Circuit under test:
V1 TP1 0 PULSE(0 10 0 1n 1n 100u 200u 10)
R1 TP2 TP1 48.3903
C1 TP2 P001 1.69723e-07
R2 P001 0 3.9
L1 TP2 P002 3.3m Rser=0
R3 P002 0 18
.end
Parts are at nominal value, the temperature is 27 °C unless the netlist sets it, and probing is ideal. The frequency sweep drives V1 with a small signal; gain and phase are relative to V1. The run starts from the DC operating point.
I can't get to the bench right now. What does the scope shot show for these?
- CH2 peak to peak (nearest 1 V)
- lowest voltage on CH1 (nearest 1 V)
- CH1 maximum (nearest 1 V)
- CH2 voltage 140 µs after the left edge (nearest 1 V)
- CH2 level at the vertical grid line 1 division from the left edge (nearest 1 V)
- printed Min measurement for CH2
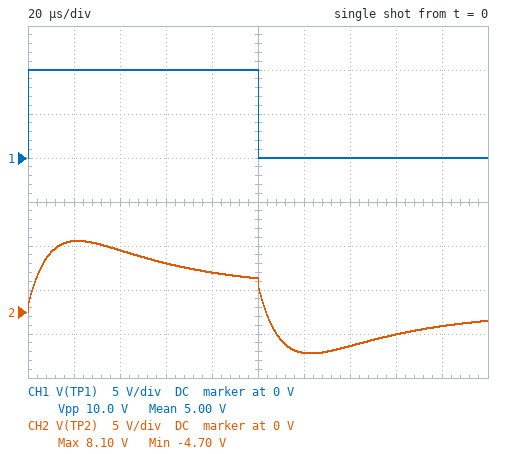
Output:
13 V
0 V
10 V
-4 V
8 V
-4.70 V
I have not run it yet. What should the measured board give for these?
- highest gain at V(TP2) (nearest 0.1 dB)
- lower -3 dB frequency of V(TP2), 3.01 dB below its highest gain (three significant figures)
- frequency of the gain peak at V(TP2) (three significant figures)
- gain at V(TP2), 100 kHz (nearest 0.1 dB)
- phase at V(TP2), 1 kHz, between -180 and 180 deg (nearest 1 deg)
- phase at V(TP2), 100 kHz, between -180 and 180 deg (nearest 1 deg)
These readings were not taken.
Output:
-0.4 dB
2.45 kHz
7.43 kHz
-14.3 dB
31 deg
-57 deg
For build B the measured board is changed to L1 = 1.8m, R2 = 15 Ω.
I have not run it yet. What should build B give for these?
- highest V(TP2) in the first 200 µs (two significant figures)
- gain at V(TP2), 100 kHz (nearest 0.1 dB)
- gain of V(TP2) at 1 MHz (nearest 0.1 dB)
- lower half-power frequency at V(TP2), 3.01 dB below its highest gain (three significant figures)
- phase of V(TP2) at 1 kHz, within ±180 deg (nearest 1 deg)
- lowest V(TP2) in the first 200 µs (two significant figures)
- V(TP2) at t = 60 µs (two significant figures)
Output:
7.0 V
-11.1 dB
-12.5 dB
3.74 kHz
22 deg
-4.3 V
3.9 V
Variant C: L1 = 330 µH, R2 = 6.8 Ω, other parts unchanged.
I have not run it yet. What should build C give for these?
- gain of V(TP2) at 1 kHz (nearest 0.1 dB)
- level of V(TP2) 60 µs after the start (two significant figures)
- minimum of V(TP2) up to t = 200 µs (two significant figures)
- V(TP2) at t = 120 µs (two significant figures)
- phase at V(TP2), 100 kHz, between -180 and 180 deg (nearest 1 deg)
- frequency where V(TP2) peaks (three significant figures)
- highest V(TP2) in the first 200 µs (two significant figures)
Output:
-11.3 dB
2.7 V
-2.3 V
-990 mV
-42 deg
22.4 kHz
5.0 V
